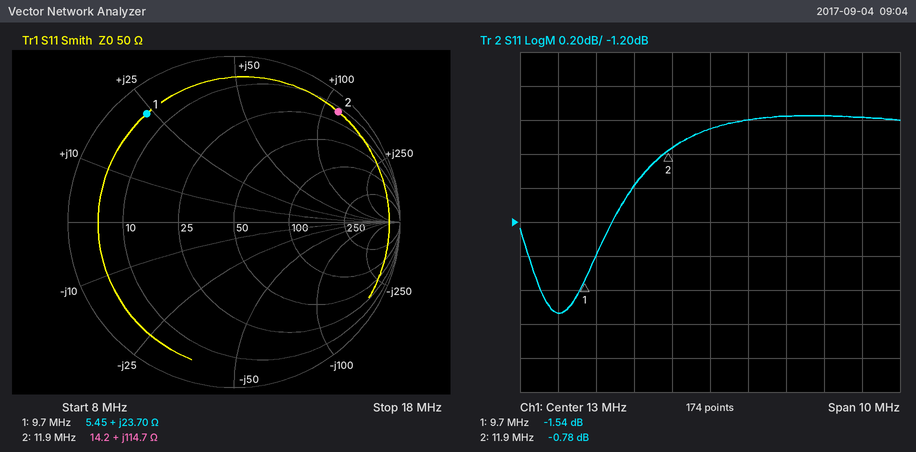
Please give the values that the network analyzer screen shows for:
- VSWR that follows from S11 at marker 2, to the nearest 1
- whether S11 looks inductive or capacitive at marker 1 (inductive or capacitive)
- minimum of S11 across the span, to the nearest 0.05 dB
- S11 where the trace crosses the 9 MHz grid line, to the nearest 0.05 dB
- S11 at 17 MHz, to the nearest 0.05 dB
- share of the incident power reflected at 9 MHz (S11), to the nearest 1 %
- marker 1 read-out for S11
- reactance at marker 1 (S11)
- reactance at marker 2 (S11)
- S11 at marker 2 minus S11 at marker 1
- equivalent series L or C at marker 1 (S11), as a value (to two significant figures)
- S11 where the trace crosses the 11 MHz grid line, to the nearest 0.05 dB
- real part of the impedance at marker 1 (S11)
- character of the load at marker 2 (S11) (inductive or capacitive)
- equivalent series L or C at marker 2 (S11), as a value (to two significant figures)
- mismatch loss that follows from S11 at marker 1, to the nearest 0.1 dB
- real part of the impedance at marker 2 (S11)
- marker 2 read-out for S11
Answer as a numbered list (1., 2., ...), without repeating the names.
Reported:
1. 22
2. inductive
3. -1.75 dB
4. -1.75 dB
5. -0.60 dB
6. 67 %
7. -1.54 dB
8. +23.70 Ω
9. +114.7 Ω
10. 0.76 dB
11. 390 nH
12. -1.00 dB
13. 5.45 Ω
14. inductive
15. 1.5 µH
16. 5.2 dB
17. 14.2 Ω
18. -0.78 dB
